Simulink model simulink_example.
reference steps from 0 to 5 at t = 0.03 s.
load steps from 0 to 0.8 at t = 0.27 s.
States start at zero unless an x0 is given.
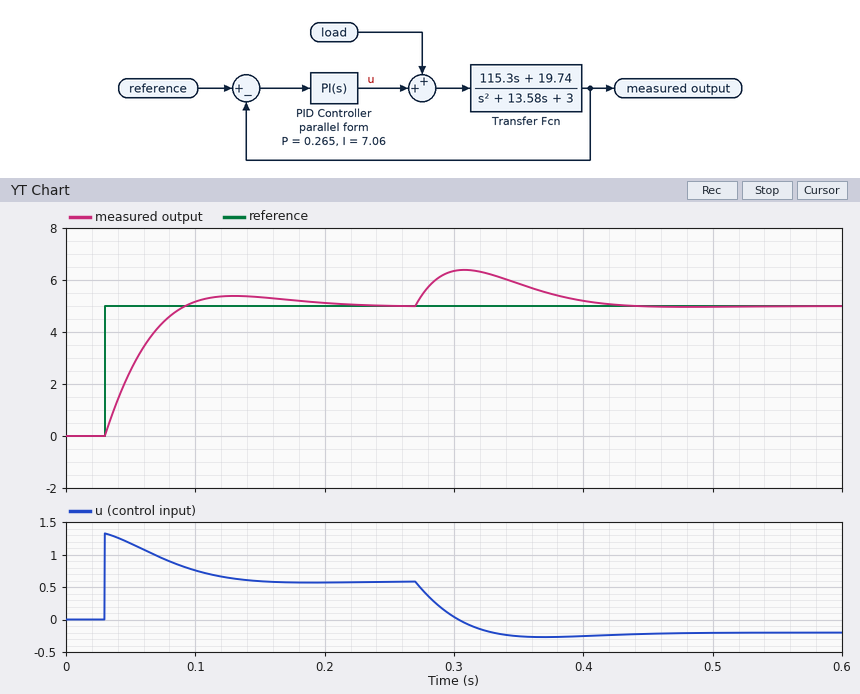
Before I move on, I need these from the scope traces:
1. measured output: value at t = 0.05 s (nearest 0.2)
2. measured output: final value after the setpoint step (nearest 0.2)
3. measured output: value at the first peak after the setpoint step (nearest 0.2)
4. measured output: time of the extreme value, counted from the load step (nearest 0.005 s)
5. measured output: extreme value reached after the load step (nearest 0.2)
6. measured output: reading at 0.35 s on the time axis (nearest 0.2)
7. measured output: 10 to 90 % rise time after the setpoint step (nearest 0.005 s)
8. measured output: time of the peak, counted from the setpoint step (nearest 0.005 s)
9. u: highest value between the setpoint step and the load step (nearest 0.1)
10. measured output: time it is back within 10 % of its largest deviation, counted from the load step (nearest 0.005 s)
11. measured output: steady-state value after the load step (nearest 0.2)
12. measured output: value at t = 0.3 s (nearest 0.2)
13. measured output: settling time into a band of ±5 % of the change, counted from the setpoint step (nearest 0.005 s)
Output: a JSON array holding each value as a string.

["2.6", "5.0", "5.4", "0.040 s", "6.4", "5.8", "0.045 s", "0.100 s", "1.3", "0.140 s", "5.0", "6.4", "0.140 s"]
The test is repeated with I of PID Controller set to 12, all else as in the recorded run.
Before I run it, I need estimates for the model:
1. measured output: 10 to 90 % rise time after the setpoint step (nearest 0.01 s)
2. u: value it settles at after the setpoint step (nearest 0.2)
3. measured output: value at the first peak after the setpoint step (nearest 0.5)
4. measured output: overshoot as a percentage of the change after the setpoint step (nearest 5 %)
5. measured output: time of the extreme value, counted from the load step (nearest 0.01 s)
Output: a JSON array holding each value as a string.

["0.03 s", "0.6", "6.0", "15 %", "0.03 s"]
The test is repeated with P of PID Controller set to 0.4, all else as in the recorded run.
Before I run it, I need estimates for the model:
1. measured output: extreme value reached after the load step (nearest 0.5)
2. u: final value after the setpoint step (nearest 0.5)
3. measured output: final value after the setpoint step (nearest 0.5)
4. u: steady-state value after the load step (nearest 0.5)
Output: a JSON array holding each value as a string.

["6.0", "0.5", "5.0", "0.0"]
